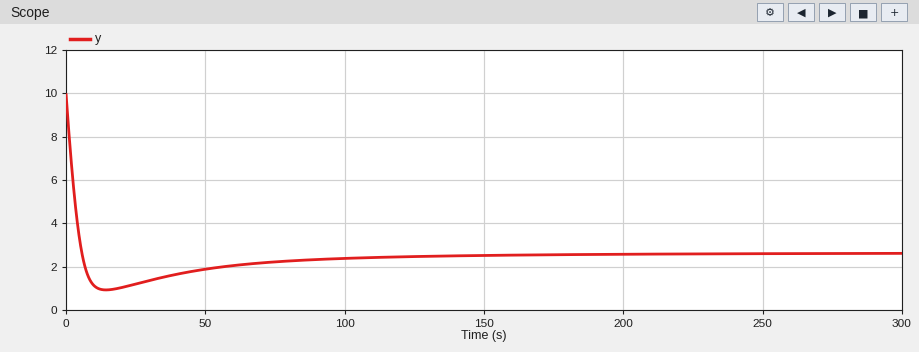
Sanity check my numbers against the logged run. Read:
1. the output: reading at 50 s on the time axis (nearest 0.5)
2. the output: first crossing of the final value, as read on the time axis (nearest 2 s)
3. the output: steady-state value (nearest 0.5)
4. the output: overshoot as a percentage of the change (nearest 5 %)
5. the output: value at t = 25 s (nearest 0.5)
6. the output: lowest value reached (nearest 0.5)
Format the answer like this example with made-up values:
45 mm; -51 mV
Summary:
2.0; 6 s; 2.5; 25 %; 1.0; 1.0
